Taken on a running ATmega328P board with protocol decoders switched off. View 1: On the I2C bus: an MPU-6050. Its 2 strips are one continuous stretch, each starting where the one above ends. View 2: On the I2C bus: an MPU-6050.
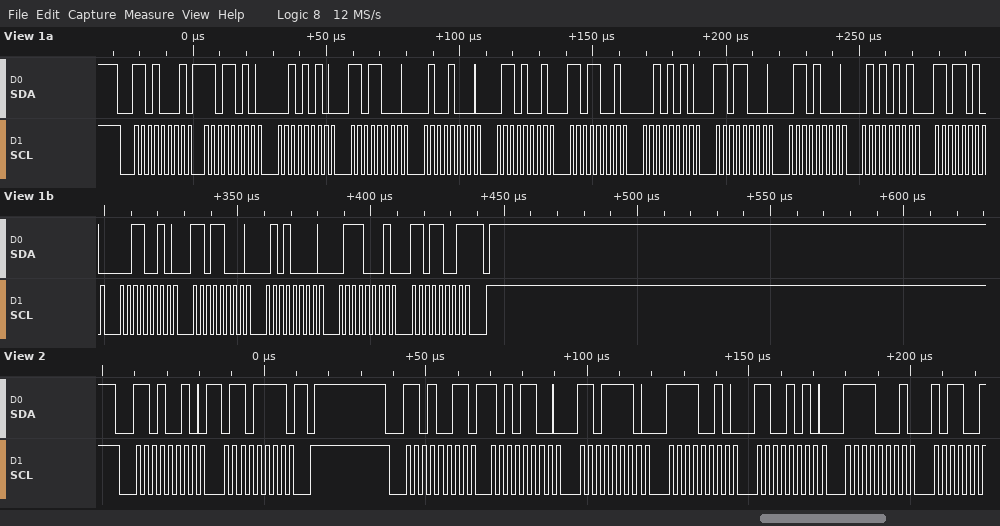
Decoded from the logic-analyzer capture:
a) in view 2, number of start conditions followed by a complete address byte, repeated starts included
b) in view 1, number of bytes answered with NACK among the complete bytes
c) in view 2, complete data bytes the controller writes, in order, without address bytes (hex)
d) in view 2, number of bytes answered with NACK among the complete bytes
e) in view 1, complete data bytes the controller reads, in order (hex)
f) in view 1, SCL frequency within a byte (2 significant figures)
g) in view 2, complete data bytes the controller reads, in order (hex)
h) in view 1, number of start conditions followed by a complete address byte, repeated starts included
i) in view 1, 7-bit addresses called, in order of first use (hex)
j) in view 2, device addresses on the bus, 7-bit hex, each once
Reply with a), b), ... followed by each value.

a) 2
b) 1
c) 6F
d) 0
e) DA 2A D8 48 69 D9 2A D8 68 55 DA 32 D8 50 71 D9
f) 400 kHz
g) AC DE F2 CA F1
h) 1
i) 0x68
j) 0x69
